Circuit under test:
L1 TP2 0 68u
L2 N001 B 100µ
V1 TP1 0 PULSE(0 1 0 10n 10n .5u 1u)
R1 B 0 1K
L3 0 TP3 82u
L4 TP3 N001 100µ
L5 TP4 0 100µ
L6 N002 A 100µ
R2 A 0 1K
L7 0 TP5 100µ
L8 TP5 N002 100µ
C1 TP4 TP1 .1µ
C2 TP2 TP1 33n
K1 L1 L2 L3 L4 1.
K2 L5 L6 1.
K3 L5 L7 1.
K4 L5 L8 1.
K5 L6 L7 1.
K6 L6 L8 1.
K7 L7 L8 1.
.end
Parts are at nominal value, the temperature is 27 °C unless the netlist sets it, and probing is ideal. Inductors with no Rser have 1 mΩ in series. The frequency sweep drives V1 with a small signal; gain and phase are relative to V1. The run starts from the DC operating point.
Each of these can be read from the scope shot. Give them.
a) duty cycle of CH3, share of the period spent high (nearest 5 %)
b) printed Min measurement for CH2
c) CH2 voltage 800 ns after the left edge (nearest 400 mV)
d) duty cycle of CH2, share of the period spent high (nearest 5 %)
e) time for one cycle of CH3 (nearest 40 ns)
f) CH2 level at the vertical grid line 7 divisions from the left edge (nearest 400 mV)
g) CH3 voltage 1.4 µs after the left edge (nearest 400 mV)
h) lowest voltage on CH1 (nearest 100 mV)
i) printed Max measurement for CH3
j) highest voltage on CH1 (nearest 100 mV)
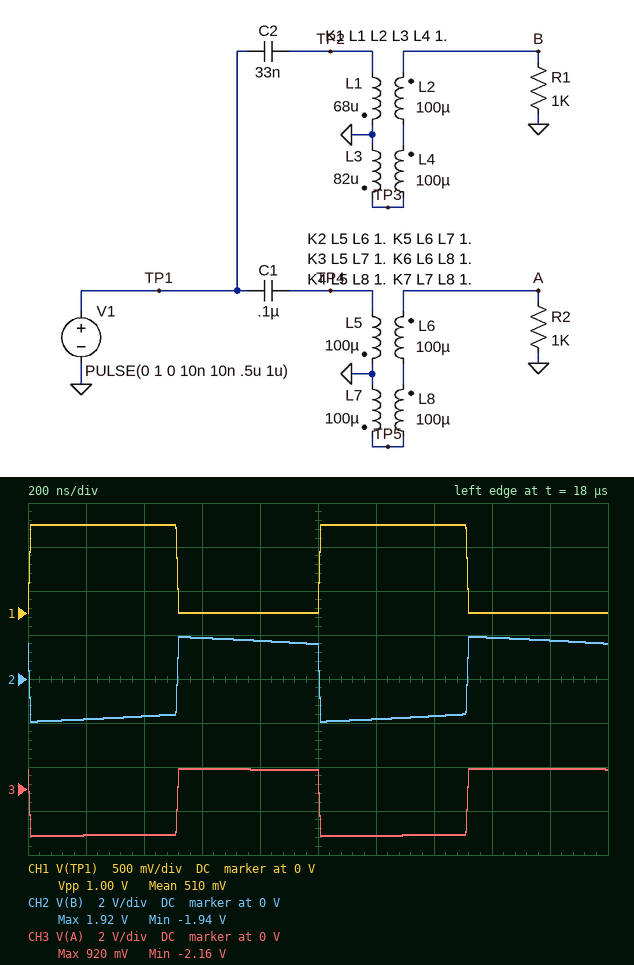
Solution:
50 %
-1.94 V
1.6 V
50 %
1.00 µs
-1.6 V
-2.0 V
0 V
920 mV
1.0 V
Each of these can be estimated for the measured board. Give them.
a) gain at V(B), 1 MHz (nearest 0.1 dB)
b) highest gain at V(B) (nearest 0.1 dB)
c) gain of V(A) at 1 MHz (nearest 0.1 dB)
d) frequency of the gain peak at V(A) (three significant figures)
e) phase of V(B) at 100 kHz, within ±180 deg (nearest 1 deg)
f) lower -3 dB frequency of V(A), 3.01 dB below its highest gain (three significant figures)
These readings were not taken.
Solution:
11.0 dB
16.3 dB
9.6 dB
51.4 kHz
-78 deg
45.2 kHz
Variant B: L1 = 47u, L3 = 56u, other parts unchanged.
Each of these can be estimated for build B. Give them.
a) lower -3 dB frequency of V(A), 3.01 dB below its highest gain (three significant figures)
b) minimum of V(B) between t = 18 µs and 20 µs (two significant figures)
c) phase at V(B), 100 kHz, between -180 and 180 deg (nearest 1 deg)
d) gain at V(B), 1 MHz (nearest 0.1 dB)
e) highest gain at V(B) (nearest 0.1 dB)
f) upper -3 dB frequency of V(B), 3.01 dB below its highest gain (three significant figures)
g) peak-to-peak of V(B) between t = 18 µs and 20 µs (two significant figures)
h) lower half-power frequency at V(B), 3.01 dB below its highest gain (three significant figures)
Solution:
45.2 kHz
-2.2 V
-51 deg
12.2 dB
16.8 dB
262 kHz
4.5 V
108 kHz
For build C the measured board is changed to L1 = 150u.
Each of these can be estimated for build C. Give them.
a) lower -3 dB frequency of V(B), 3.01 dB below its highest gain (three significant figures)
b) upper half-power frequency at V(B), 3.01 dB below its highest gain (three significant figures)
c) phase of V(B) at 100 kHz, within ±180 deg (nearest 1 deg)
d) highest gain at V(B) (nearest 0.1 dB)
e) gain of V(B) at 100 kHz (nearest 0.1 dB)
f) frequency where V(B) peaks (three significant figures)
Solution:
62.7 kHz
96.0 kHz
-151 deg
16.1 dB
12.6 dB
74.3 kHz
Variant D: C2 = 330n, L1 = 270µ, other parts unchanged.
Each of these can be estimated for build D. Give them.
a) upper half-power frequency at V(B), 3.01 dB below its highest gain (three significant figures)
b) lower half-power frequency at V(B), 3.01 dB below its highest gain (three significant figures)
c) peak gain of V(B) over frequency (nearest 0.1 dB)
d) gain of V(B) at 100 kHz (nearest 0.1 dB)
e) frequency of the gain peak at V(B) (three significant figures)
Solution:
17.7 kHz
16.2 kHz
25.9 dB
5.2 dB
16.9 kHz
